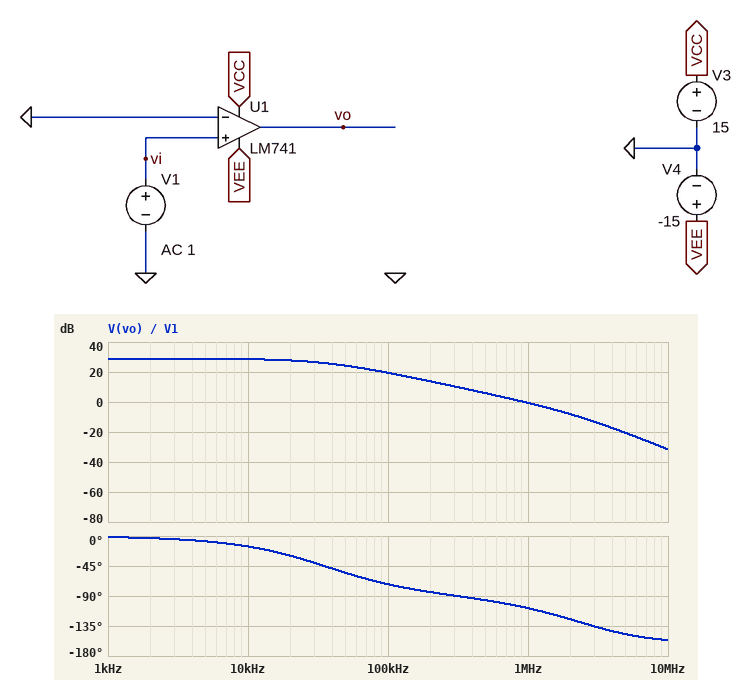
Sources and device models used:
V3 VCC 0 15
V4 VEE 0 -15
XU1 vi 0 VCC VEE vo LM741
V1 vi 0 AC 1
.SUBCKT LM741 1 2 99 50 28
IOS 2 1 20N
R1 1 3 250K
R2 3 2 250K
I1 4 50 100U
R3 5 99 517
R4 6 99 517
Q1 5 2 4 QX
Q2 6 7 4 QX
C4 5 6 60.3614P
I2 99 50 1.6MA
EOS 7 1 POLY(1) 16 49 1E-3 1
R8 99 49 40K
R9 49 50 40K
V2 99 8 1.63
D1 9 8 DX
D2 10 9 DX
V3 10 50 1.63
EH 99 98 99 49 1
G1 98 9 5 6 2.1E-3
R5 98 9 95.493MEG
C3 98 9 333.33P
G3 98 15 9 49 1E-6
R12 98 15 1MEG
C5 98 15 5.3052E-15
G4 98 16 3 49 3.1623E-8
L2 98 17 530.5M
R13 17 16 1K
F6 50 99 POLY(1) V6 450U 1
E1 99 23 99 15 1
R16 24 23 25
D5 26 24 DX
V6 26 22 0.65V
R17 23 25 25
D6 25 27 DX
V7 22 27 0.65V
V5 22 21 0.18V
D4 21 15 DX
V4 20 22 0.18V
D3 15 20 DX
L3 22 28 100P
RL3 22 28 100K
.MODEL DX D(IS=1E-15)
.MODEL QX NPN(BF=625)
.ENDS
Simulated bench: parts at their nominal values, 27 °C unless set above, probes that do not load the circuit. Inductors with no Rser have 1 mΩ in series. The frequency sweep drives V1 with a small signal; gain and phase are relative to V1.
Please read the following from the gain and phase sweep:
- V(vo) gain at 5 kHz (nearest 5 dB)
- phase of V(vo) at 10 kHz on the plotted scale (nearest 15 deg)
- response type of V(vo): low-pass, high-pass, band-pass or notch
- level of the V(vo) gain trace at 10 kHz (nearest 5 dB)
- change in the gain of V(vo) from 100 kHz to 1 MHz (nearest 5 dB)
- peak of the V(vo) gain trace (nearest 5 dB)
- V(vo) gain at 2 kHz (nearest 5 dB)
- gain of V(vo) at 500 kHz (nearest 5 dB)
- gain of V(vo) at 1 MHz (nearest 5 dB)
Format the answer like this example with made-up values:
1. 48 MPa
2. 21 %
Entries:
1. 30 dB
2. -15 deg
3. low-pass
4. 30 dB
5. -20 dB
6. 30 dB
7. 30 dB
8. 5 dB
9. 0 dB
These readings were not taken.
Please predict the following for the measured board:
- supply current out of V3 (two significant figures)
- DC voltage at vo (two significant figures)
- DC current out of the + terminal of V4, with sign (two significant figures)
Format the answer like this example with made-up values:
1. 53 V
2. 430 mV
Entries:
1. 1.7 mA
2. 14 V
3. -1.7 mA
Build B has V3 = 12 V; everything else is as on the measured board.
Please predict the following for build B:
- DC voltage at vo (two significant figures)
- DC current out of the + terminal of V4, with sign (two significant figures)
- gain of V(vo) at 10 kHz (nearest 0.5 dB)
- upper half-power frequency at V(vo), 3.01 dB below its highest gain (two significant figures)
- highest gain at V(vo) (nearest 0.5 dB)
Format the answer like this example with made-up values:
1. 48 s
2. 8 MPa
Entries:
1. 11 V
2. -1.7 mA
3. 28.0 dB
4. 38 kHz
5. 28.5 dB
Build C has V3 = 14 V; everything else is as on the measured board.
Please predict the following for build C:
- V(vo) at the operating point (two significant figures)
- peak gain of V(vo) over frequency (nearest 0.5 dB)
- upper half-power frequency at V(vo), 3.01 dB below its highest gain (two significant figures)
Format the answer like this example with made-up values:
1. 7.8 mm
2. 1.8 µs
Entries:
1. 13 V
2. 28.5 dB
3. 37 kHz
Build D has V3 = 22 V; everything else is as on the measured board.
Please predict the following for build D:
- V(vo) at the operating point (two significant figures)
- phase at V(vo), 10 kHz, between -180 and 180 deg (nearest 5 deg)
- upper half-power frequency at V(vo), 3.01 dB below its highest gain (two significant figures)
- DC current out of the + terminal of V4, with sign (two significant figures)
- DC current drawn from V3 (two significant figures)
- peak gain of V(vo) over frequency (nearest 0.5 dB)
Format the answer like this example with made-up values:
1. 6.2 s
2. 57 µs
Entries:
1. 21 V
2. -20 deg
3. 31 kHz
4. -1.8 mA
5. 1.8 mA
6. 30.0 dB
